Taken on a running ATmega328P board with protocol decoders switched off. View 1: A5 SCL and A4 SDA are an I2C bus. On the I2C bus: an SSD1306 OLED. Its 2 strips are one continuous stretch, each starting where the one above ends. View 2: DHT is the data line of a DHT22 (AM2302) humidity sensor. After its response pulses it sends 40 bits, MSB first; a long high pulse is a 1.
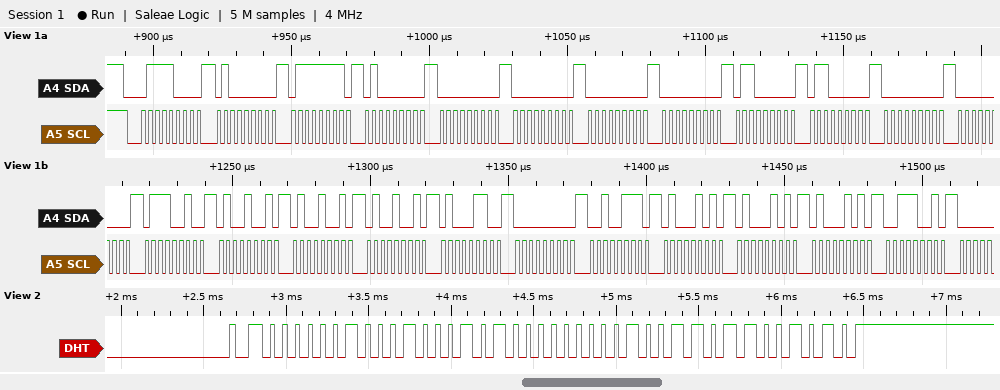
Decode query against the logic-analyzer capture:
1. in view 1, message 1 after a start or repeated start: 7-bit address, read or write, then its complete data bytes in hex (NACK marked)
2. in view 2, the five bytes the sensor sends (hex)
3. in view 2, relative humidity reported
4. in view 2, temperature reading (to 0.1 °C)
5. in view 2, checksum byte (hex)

0x3C write: 40 7F 40 00 00 00 00 60 60 00 00 72 49 49 49 46 00 27 45 45 45 39
02 22 80 26 CA
54.6 %
-3.8 °C
0xCA
